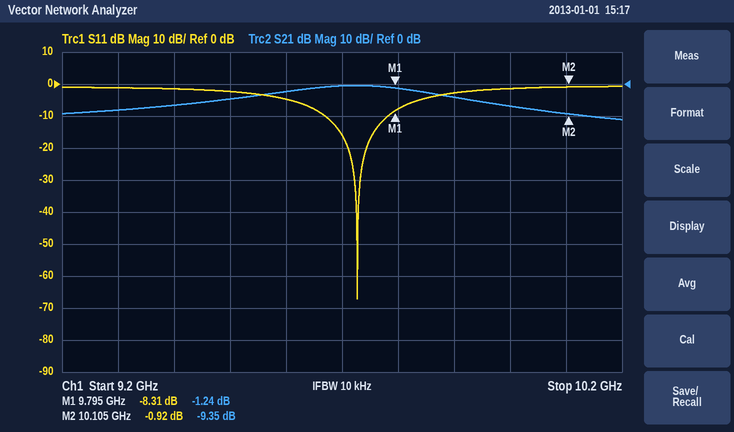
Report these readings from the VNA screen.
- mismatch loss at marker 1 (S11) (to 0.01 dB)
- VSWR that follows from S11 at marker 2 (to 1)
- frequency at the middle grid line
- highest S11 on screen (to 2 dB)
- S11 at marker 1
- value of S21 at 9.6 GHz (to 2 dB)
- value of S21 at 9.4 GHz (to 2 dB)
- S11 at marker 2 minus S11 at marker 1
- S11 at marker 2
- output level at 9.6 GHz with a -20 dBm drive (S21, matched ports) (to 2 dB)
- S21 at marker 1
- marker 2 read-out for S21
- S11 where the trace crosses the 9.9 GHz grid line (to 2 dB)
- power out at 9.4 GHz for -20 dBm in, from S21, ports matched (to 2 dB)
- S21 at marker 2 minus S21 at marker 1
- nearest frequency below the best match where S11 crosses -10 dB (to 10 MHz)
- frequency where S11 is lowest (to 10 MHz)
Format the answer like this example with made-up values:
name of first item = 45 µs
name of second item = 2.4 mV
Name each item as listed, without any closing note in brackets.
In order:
mismatch loss at marker 1 (S11) = 0.69 dB
VSWR that follows from S11 at marker 2 = 19
frequency at the middle grid line = 9.7 GHz
highest S11 on screen = 0 dB
S11 at marker 1 = -8.31 dB
value of S21 at 9.6 GHz = -2 dB
value of S21 at 9.4 GHz = -6 dB
S11 at marker 2 minus S11 at marker 1 = 7.39 dB
S11 at marker 2 = -0.92 dB
output level at 9.6 GHz with a -20 dBm drive (S21, matched ports) = -22 dBm
S21 at marker 1 = -1.24 dB
marker 2 read-out for S21 = -9.35 dB
S11 where the trace crosses the 9.9 GHz grid line = -2 dB
power out at 9.4 GHz for -20 dBm in, from S21, ports matched = -26 dBm
S21 at marker 2 minus S21 at marker 1 = -8.11 dB
nearest frequency below the best match where S11 crosses -10 dB = 9.67 GHz
frequency where S11 is lowest = 9.73 GHz
